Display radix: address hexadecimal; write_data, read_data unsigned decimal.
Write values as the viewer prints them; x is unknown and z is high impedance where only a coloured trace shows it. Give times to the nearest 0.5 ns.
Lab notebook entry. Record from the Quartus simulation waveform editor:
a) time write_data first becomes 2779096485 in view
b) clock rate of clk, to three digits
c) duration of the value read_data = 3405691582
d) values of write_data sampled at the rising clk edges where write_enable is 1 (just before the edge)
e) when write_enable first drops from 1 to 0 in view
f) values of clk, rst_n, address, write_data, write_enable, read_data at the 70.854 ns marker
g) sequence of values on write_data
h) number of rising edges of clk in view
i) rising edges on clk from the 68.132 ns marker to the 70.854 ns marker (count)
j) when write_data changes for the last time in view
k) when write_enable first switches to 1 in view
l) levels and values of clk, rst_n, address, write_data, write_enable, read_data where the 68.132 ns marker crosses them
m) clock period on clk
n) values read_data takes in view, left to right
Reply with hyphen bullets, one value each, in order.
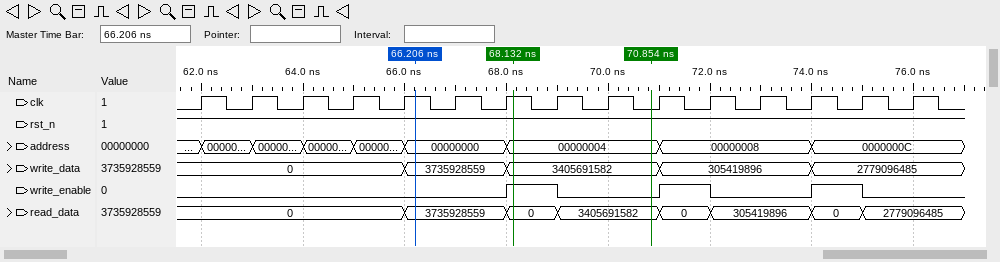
- 74 ns
- 1.00 GHz
- 2 ns
- 3405691582, 305419896, 2779096485
- 69 ns
- clk=0, rst_n=1, address=00000004, write_data=3405691582, write_enable=0, read_data=3405691582
- 0, 3735928559, 3405691582, 305419896, 2779096485
- 15
- 2
- 74 ns
- 68 ns
- clk=1, rst_n=1, address=00000004, write_data=3405691582, write_enable=1, read_data=0
- 1 ns
- 0, 3735928559, 0, 3405691582, 0, 305419896, 0, 2779096485
